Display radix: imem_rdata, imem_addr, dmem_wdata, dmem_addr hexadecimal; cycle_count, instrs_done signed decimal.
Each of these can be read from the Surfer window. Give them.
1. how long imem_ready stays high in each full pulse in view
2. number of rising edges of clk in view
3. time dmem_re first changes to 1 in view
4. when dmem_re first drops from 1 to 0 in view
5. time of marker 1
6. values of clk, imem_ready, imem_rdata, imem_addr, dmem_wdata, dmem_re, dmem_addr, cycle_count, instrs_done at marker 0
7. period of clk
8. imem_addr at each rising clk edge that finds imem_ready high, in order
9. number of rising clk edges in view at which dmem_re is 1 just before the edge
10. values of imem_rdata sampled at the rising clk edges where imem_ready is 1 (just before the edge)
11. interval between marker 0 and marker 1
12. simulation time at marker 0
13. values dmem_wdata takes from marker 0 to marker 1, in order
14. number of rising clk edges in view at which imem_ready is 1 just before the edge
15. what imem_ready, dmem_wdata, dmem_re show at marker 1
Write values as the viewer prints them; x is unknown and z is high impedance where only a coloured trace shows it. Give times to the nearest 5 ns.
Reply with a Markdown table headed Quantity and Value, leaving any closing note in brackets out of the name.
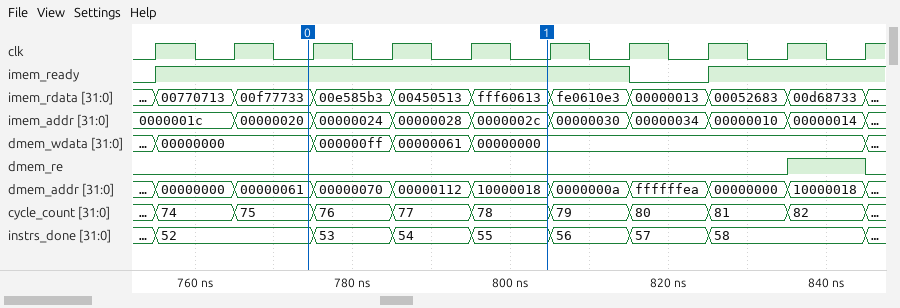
| Quantity | Value |
|---|---|
| how long imem_ready stays high in each full pulse in view | 60 ns |
| number of rising edges of clk in view | 10 |
| time dmem_re first changes to 1 in view | 835 ns |
| when dmem_re first drops from 1 to 0 in view | 845 ns |
| time of marker 1 | 805 ns |
| values of clk, imem_ready, imem_rdata, imem_addr, dmem_wdata, dmem_re, dmem_addr, cycle_count, instrs_done at marker 0 | clk=0, imem_ready=1, imem_rdata=00f77733, imem_addr=00000020, dmem_wdata=00000000, dmem_re=0, dmem_addr=00000061, cycle_count=75, instrs_done=52 |
| period of clk | 10 ns |
| imem_addr at each rising clk edge that finds imem_ready high, in order | 0000001c, 00000020, 00000024, 00000028, 0000002c, 00000030, 00000010, 00000014 |
| number of rising clk edges in view at which dmem_re is 1 just before the edge | 1 |
| values of imem_rdata sampled at the rising clk edges where imem_ready is 1 | 00770713, 00f77733, 00e585b3, 00450513, fff60613, fe0610e3, 00052683, 00d68733 |
| interval between marker 0 and marker 1 | 30 ns |
| simulation time at marker 0 | 775 ns |
| values dmem_wdata takes from marker 0 to marker 1, in order | 00000000, 000000ff, 00000061, 00000000 |
| number of rising clk edges in view at which imem_ready is 1 just before the edge | 8 |
| what imem_ready, dmem_wdata, dmem_re show at marker 1 | imem_ready=1, dmem_wdata=00000000, dmem_re=0 |
